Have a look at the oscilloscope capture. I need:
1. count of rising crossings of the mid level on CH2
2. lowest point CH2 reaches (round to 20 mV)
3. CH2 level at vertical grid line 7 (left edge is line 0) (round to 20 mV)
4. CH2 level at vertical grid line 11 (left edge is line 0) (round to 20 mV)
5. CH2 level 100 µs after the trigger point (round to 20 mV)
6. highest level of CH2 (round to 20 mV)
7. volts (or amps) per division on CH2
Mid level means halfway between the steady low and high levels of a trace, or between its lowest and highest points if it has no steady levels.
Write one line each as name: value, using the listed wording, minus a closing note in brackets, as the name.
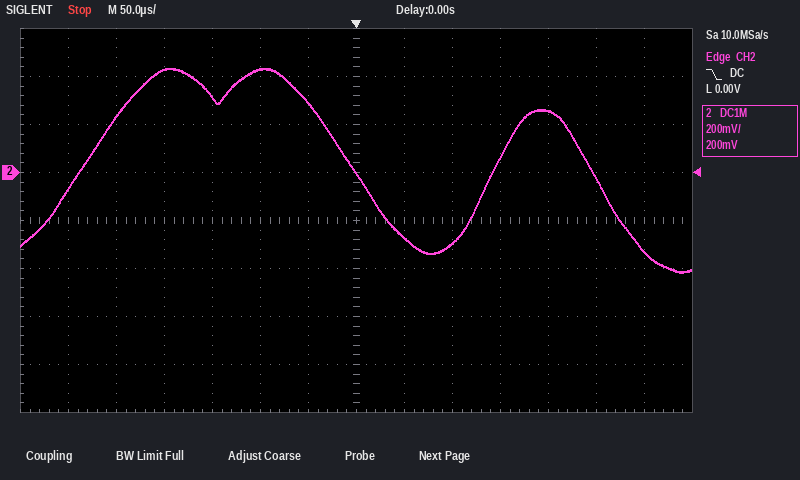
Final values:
count of rising crossings of the mid level on CH2: 2
lowest point CH2 reaches: -420 mV
CH2 level at vertical grid line 7 (left edge is line 0): 0 mV
CH2 level at vertical grid line 11 (left edge is line 0): 260 mV
CH2 level 100 µs after the trigger point: -300 mV
highest level of CH2: 440 mV
volts (or amps) per division on CH2: 200 mV
